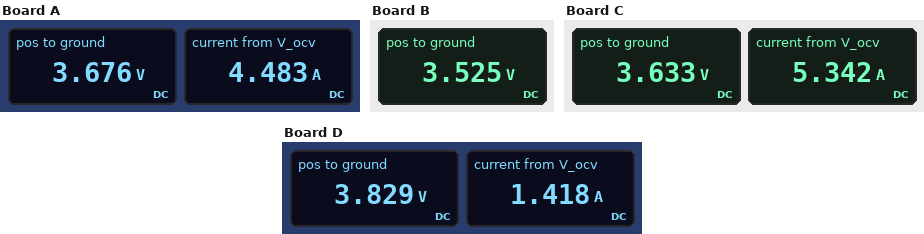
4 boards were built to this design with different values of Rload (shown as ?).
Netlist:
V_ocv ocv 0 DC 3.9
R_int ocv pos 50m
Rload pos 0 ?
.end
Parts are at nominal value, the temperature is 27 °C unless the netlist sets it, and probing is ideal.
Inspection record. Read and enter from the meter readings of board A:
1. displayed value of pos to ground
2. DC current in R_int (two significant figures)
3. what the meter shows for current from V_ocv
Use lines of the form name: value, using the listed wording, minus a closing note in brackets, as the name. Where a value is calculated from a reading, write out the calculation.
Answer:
displayed value of pos to ground: 3.676 V
DC current in R_int: (3.9 V - 3.676 V) / 50 mΩ = 4.5 A
what the meter shows for current from V_ocv: 4.483 A
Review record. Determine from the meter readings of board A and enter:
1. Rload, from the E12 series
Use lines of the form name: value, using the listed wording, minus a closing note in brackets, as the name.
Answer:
Rload, from the E12 series: 0.82 Ω
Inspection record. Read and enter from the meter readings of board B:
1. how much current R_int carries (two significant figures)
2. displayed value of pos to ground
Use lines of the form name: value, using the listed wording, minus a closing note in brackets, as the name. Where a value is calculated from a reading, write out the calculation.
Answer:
how much current R_int carries: (3.9 V - 3.525 V) / 50 mΩ = 7.5 A
displayed value of pos to ground: 3.525 V
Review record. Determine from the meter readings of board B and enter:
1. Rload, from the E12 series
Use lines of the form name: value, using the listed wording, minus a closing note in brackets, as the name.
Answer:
Rload, from the E12 series: 0.47 Ω
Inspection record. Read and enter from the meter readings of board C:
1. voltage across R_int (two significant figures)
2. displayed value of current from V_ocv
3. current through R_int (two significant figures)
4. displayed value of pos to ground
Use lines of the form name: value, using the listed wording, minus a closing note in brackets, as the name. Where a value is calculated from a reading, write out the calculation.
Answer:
voltage across R_int: 3.9 V - 3.633 V = 270 mV
displayed value of current from V_ocv: 5.342 A
current through R_int: (3.9 V - 3.633 V) / 50 mΩ = 5.3 A
displayed value of pos to ground: 3.633 V
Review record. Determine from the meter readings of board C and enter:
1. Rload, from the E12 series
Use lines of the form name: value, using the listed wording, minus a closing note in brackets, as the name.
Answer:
Rload, from the E12 series: 0.68 Ω
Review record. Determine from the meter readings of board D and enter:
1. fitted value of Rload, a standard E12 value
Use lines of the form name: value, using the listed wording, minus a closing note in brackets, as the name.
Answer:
fitted value of Rload, a standard E12 value: 2.7 Ω
